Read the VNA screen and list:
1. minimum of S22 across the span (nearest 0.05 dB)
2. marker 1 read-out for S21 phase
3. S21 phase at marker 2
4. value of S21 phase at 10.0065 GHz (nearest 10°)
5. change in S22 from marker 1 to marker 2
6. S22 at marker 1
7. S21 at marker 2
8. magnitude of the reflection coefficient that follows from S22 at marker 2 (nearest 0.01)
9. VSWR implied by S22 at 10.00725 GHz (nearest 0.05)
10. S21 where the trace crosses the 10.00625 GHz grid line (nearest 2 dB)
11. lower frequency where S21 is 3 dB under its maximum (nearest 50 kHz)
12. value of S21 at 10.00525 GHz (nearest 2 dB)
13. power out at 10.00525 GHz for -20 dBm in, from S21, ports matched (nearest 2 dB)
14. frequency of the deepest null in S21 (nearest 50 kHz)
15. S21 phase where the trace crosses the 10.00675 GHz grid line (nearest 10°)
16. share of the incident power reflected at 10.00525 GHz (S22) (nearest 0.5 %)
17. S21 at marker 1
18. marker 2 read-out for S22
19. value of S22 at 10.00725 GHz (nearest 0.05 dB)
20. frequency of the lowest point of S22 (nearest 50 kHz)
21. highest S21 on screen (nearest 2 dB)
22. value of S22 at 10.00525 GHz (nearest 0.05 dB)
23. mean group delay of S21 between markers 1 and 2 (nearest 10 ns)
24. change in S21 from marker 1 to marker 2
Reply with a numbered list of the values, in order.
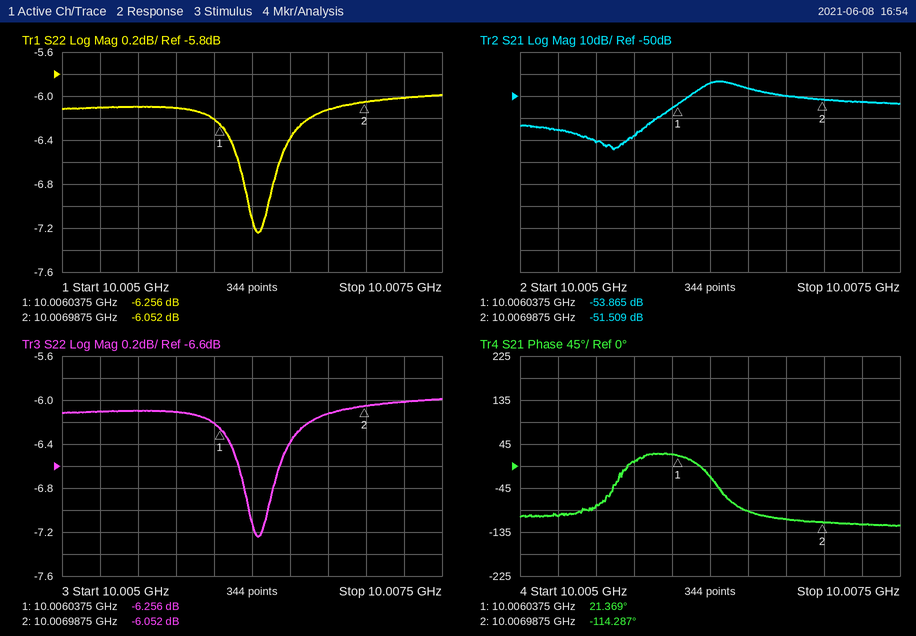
1. -7.25 dB
2. 21.369°
3. -114.287°
4. -90°
5. 0.204 dB
6. -6.256 dB
7. -51.509 dB
8. 0.50
9. 3.00
10. -44 dB
11. 10.00620 GHz
12. -66 dB
13. -86 dBm
14. 10.00560 GHz
15. -110°
16. 24.5 %
17. -53.865 dB
18. -6.052 dB
19. -6.00 dB
20. 10.00630 GHz
21. -44 dB
22. -6.10 dB
23. 400 ns
24. 2.356 dB
